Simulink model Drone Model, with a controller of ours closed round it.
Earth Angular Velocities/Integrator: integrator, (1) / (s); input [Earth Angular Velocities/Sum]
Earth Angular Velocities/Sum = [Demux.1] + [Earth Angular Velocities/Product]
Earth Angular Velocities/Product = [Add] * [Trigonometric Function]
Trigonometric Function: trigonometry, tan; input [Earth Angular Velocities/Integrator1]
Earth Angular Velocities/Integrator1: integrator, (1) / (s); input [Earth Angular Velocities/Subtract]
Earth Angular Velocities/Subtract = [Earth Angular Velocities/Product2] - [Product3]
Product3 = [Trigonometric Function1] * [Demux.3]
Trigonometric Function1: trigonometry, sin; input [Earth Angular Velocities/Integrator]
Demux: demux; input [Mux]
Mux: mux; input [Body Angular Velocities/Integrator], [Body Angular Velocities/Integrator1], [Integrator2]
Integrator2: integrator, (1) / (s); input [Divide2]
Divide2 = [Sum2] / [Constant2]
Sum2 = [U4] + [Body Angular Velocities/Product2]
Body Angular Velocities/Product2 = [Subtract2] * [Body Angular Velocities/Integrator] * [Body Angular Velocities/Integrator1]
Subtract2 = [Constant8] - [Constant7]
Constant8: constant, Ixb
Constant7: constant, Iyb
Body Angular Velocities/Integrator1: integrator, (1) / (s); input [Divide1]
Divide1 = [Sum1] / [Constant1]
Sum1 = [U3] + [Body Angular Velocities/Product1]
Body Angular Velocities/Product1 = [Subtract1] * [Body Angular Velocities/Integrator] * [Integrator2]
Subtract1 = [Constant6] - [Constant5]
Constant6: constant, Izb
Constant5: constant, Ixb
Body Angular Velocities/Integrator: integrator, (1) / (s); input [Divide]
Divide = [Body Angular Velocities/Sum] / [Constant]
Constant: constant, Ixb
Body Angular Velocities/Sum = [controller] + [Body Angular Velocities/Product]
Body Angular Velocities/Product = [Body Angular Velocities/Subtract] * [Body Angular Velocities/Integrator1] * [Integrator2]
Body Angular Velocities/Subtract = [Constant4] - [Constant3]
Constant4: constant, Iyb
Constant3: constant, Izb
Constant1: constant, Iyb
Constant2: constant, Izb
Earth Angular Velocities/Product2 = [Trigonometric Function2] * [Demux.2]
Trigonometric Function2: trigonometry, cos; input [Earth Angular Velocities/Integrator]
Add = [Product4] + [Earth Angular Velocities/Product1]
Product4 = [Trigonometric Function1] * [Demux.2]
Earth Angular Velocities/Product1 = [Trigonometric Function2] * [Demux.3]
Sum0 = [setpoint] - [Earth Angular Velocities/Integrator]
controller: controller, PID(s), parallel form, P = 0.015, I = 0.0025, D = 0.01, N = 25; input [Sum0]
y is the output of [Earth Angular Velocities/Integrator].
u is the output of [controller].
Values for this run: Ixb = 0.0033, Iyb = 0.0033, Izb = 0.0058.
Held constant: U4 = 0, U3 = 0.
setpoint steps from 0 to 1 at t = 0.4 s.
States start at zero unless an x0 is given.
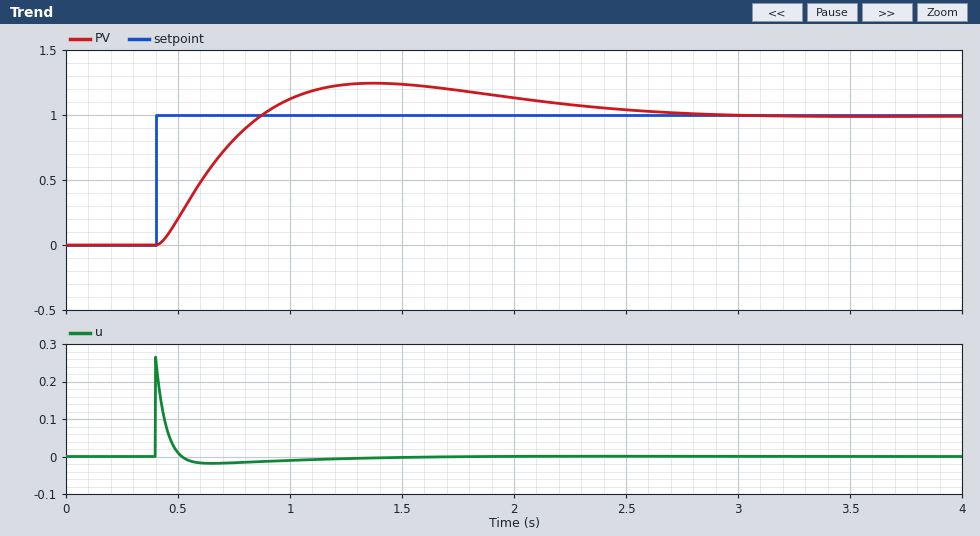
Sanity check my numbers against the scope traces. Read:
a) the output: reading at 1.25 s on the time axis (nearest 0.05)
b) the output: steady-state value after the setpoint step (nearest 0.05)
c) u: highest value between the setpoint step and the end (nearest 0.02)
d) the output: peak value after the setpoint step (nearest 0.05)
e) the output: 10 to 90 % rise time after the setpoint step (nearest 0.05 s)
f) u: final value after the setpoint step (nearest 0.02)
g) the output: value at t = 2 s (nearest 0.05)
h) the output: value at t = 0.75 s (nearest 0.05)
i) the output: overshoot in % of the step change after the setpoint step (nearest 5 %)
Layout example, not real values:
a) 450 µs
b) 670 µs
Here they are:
a) 1.25
b) 1.00
c) 0.26
d) 1.25
e) 0.35 s
f) 0.00
g) 1.15
h) 0.80
i) 25 %
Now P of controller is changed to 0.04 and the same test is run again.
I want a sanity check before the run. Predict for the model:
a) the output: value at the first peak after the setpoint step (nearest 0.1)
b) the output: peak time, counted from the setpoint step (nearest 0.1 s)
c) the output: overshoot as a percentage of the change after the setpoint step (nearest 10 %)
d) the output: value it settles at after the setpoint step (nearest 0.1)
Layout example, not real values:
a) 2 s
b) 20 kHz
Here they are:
a) 1.4
b) 0.7 s
c) 40 %
d) 1.0
